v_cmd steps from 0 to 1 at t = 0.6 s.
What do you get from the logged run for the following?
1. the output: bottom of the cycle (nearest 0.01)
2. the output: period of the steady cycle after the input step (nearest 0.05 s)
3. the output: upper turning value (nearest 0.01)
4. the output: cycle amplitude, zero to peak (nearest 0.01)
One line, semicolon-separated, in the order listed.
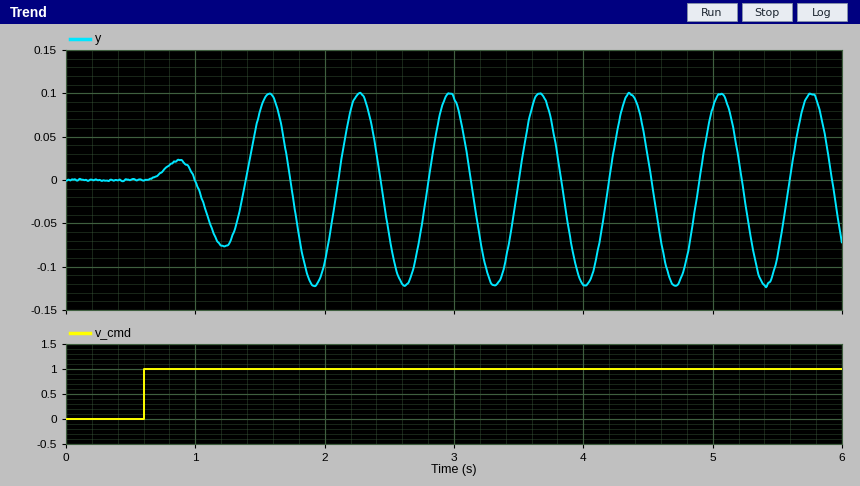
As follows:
-0.12; 0.70 s; 0.10; 0.11
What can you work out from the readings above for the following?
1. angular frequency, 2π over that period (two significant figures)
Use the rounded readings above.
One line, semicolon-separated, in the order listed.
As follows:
9.0 rad/s
